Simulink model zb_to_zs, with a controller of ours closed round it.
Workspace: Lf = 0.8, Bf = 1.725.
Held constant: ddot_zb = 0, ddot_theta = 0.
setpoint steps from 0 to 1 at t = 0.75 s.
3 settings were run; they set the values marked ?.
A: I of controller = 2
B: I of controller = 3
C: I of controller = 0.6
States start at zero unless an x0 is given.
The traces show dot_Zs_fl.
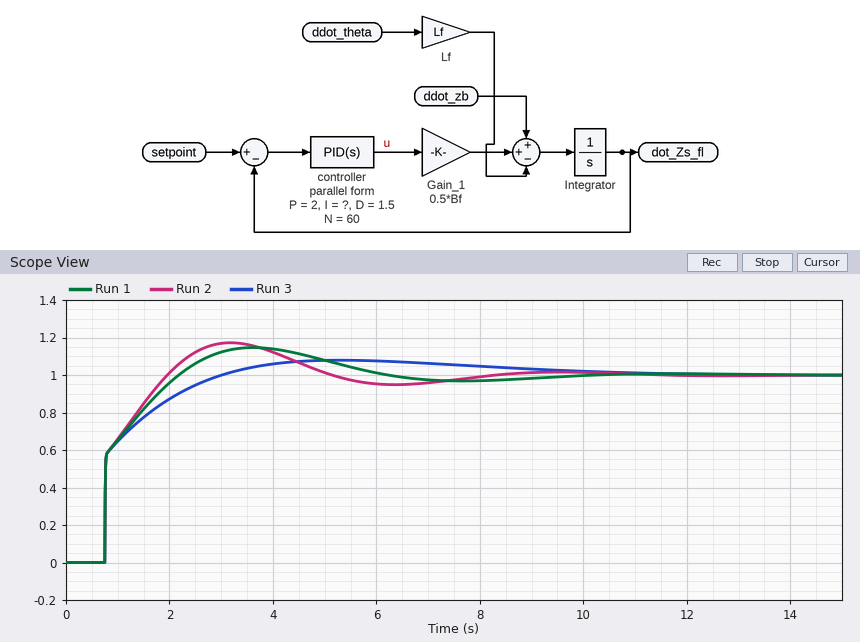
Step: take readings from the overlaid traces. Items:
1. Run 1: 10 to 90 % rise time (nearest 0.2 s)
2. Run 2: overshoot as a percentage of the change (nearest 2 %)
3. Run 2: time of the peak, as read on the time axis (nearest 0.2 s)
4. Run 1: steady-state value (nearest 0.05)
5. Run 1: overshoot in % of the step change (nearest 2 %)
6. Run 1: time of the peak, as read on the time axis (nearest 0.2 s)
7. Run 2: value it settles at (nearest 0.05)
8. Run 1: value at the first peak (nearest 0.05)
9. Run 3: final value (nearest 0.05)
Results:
1.0 s
18 %
3.2 s
1.00
14 %
3.6 s
1.00
1.15
1.00
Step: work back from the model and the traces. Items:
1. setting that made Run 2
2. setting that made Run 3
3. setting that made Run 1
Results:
B
C
A
